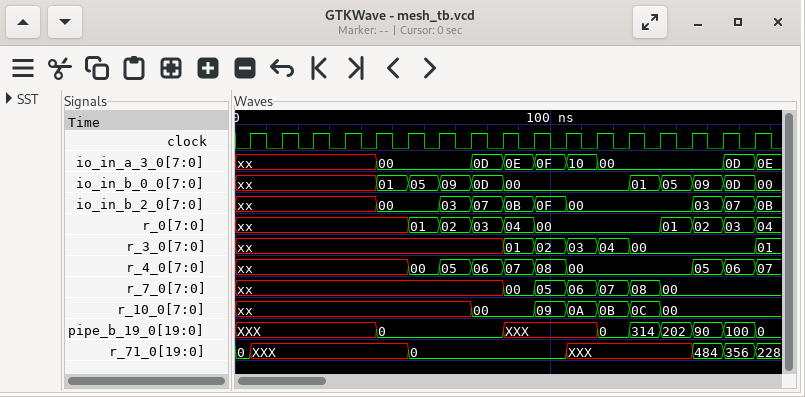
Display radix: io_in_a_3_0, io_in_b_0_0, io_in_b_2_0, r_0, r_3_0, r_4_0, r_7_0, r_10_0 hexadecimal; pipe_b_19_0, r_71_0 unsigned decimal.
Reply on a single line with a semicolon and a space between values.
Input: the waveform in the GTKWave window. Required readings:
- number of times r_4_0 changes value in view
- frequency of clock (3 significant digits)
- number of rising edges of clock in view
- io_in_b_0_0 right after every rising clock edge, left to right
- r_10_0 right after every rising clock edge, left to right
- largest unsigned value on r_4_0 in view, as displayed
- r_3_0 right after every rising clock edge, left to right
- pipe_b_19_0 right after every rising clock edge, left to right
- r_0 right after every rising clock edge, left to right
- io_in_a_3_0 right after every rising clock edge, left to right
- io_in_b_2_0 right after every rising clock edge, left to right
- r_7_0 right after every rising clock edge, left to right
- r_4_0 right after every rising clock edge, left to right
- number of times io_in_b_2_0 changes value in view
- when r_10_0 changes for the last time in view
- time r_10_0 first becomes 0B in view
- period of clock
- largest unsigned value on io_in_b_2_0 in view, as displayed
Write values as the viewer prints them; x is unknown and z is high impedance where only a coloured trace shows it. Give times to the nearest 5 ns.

9; 100 MHz; 17; xx, xx, xx, xx, 01, 05, 09, 0D, 00, 00, 00, 00, 01, 05, 09, 0D, 00; xx, xx, xx, xx, xx, xx, xx, 00, 00, 09, 0A, 0B, 0C, 00, 00, 00, 00; 08; xx, xx, xx, xx, xx, xx, xx, xx, 01, 02, 03, 04, 00, 00, 00, 00, 01; XXX, XXX, XXX, XXX, 0, 0, 0, 0, XXX, XXX, XXX, 0, 314, 202, 90, 100, 0; xx, xx, xx, xx, xx, 01, 02, 03, 04, 00, 00, 00, 00, 01, 02, 03, 04; xx, xx, xx, xx, 00, 00, 00, 0D, 0E, 0F, 10, 00, 00, 00, 00, 0D, 0E; xx, xx, xx, xx, 00, 00, 03, 07, 0B, 0F, 00, 00, 00, 00, 03, 07, 0B; xx, xx, xx, xx, xx, xx, xx, xx, 00, 05, 06, 07, 08, 00, 00, 00, 00; xx, xx, xx, xx, xx, 00, 05, 06, 07, 08, 00, 00, 00, 00, 05, 06, 07; 9; 135 ns; 115 ns; 10 ns; 0F
